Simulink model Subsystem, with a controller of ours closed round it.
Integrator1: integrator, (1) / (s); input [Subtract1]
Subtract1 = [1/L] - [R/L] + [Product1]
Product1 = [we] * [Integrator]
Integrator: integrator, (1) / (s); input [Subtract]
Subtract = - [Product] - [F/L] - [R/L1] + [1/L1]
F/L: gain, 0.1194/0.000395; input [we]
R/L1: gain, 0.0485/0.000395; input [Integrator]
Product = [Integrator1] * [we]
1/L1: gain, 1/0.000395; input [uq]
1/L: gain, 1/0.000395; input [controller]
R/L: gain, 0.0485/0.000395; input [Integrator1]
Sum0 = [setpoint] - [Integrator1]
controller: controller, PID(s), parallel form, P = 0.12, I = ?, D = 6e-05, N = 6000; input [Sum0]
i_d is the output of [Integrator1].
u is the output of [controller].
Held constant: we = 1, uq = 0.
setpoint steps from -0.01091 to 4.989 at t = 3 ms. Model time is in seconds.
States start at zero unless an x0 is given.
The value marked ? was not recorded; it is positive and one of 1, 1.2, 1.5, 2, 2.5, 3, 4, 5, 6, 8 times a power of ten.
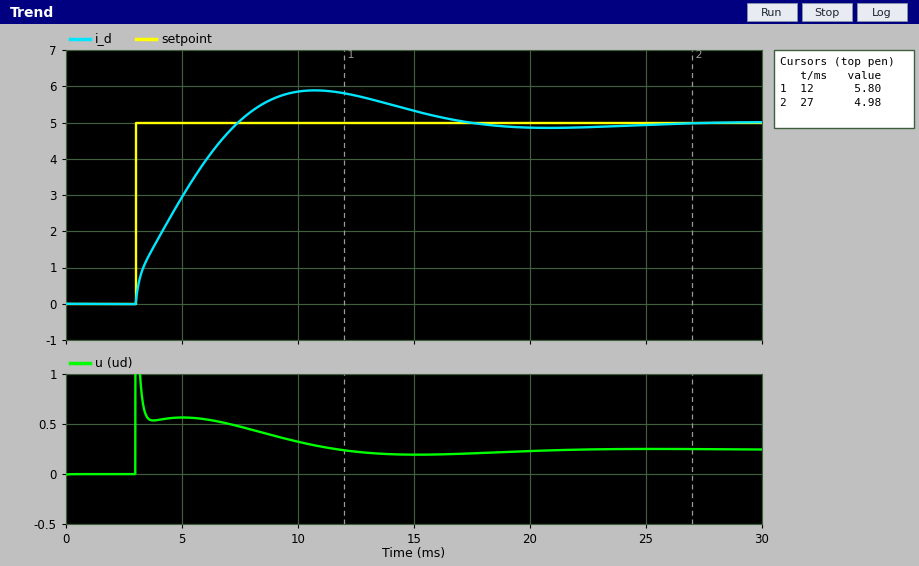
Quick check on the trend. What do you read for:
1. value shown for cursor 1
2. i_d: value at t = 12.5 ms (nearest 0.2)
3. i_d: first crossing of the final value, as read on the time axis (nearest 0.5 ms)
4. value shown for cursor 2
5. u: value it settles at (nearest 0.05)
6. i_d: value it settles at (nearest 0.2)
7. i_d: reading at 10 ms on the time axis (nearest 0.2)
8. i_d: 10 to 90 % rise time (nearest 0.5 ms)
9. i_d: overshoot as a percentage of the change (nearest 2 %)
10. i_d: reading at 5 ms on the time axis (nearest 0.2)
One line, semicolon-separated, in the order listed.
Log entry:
5.80; 5.8; 7.5 ms; 4.98; 0.25; 5.0; 5.8; 3.5 ms; 18 %; 3.0
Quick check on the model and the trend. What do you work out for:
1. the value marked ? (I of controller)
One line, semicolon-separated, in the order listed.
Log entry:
60
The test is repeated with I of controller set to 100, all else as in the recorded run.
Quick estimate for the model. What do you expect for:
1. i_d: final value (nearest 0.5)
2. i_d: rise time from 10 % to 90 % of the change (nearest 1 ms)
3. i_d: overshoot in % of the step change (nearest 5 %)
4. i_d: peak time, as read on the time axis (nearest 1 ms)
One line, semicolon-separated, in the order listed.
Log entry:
5.0; 3 ms; 25 %; 9 ms
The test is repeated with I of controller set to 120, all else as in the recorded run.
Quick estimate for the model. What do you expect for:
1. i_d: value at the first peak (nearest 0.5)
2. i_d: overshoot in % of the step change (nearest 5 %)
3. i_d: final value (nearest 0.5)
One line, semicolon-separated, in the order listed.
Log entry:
6.5; 30 %; 5.0
